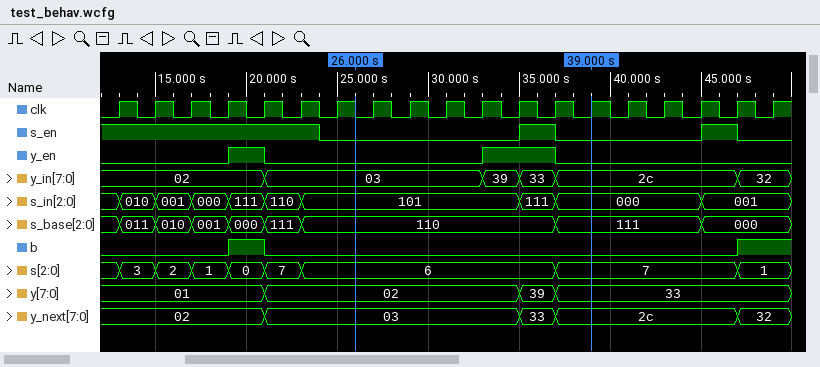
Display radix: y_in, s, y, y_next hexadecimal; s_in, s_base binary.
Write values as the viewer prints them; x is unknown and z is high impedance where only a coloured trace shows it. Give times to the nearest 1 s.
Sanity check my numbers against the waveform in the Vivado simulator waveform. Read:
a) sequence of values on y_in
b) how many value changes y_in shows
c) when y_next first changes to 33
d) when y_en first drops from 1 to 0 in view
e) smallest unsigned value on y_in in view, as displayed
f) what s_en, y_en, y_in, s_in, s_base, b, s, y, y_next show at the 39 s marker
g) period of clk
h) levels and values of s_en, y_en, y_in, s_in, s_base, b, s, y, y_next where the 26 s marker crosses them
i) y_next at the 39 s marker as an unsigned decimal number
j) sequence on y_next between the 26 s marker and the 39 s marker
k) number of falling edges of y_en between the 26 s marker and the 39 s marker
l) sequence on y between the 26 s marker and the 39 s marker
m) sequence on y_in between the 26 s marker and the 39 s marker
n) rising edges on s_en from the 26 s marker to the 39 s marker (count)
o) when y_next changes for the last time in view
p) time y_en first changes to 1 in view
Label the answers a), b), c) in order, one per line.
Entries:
a) 02, 03, 39, 33, 2c, 32
b) 5
c) 35 s
d) 21 s
e) 02
f) s_en=0, y_en=0, y_in=2c, s_in=000, s_base=111, b=0, s=7, y=33, y_next=2c
g) 2 s
h) s_en=0, y_en=0, y_in=03, s_in=101, s_base=110, b=0, s=6, y=02, y_next=03
i) 44
j) 03, 33, 2c
k) 1
l) 02, 39, 33
m) 03, 39, 33, 2c
n) 1
o) 47 s
p) 19 s
